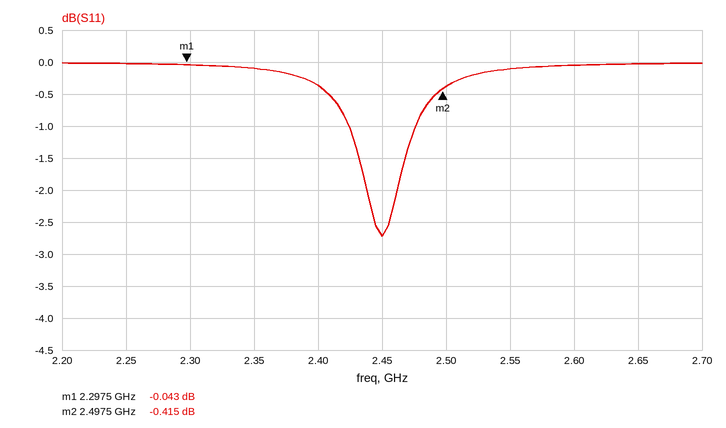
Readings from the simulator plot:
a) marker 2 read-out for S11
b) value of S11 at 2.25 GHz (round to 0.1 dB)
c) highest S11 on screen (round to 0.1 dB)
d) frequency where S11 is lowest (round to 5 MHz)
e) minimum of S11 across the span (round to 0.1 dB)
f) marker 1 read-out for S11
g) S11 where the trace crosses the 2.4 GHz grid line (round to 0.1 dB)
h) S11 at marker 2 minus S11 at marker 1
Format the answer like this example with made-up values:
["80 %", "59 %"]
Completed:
["-0.415 dB", "0.0 dB", "0.0 dB", "2.450 GHz", "-2.7 dB", "-0.043 dB", "-0.4 dB", "-0.372 dB"]
